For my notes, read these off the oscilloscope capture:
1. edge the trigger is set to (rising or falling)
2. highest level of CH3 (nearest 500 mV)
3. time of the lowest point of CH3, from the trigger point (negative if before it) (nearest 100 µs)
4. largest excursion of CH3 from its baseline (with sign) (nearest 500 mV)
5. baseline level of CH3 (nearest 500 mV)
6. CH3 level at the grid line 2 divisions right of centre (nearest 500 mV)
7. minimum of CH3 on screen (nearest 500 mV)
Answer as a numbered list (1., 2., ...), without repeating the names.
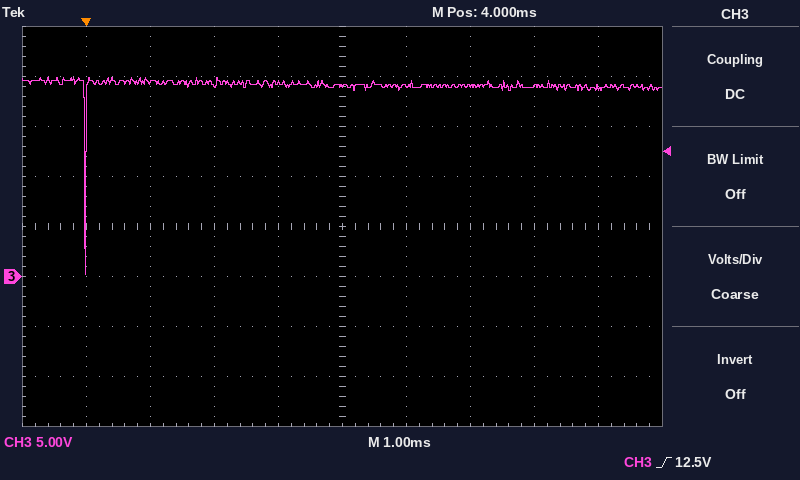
1. rising
2. 20.0 V
3. 0.0 ms
4. -19.0 V
5. 19.0 V
6. 19.0 V
7. 0.0 V
